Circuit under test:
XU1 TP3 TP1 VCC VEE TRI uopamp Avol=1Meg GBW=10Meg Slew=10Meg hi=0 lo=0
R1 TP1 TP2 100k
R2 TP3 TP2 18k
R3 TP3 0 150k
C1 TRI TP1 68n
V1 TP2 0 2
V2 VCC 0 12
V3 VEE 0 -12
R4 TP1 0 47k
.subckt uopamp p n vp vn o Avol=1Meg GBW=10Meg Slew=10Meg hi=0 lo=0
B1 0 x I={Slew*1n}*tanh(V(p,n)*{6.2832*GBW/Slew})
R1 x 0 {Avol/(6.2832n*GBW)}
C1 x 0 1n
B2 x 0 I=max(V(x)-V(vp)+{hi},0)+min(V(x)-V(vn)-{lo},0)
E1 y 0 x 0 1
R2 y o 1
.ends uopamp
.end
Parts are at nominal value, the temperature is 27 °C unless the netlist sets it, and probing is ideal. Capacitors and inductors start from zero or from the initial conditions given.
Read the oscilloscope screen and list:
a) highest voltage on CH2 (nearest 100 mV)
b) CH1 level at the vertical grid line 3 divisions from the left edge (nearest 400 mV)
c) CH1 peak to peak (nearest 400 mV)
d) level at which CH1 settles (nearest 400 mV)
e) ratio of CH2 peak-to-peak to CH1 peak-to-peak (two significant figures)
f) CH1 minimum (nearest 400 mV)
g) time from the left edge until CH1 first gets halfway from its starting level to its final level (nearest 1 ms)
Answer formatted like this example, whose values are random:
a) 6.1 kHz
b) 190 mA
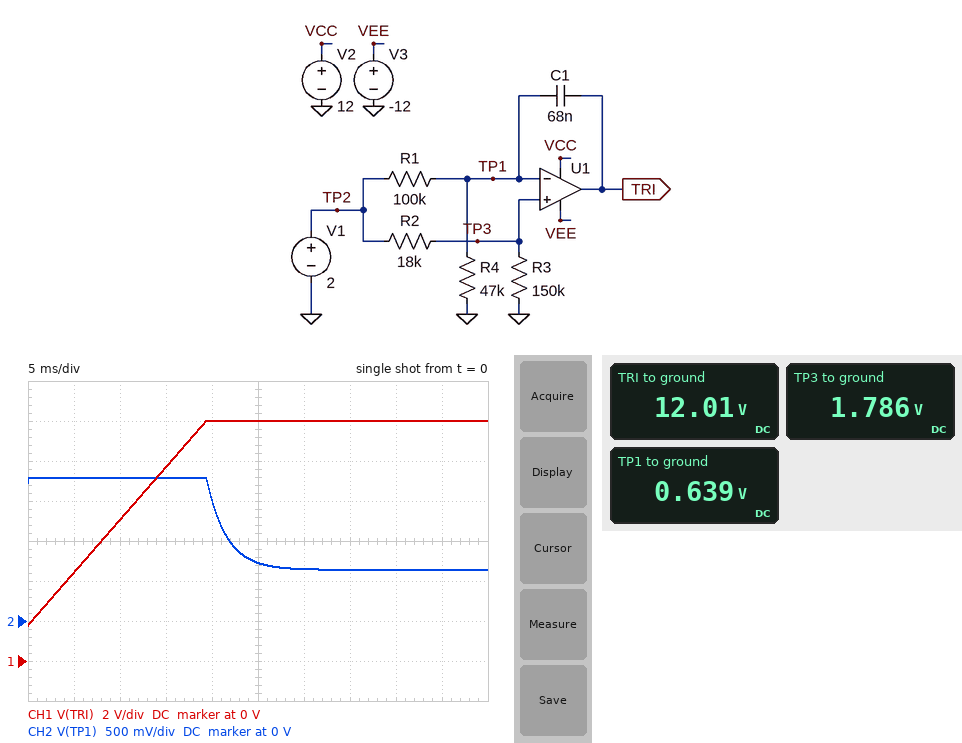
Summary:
a) 1.8 V
b) 9.6 V
c) 10.4 V
d) 12.0 V
e) 0.11
f) 1.6 V
g) 10 ms
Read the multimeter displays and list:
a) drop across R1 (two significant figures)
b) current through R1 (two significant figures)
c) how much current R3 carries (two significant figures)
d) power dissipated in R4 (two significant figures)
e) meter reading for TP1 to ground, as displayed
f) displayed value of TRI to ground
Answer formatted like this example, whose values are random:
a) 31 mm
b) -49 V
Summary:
a) 1.4 V
b) 14 µA
c) 12 µA
d) 8.7 µW
e) 0.639 V
f) 12.01 V
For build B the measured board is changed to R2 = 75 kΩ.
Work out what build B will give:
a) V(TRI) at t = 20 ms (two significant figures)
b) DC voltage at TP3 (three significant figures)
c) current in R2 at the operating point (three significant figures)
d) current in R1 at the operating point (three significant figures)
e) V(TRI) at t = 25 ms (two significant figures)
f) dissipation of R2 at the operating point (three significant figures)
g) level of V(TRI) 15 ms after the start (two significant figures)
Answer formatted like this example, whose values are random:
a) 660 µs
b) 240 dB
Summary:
a) 7.7 V
b) 1.33 V
c) 8.89 µA
d) 13.6 µA
e) 9.3 V
f) 5.93 µW
g) 6.1 V
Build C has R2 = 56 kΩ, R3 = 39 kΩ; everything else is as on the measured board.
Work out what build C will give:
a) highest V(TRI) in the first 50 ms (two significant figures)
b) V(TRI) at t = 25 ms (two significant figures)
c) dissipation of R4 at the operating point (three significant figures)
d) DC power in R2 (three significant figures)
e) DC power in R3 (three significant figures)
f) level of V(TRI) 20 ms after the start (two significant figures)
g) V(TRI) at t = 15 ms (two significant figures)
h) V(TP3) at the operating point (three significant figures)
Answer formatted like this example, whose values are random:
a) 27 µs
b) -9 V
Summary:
a) 5.0 V
b) 2.9 V
c) 8.70 µW
d) 24.8 µW
e) 17.3 µW
f) 2.5 V
g) 2.1 V
h) 821 mV
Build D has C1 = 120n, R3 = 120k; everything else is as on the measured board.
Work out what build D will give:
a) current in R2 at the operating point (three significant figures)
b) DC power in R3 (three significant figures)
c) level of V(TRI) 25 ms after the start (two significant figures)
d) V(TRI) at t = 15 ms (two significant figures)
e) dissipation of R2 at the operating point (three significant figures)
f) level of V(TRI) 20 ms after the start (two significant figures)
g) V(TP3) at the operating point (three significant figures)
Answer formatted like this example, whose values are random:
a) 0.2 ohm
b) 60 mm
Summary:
a) 14.5 µA
b) 25.2 µW
c) 8.9 V
d) 6.0 V
e) 3.78 µW
f) 7.5 V
g) 1.74 V
